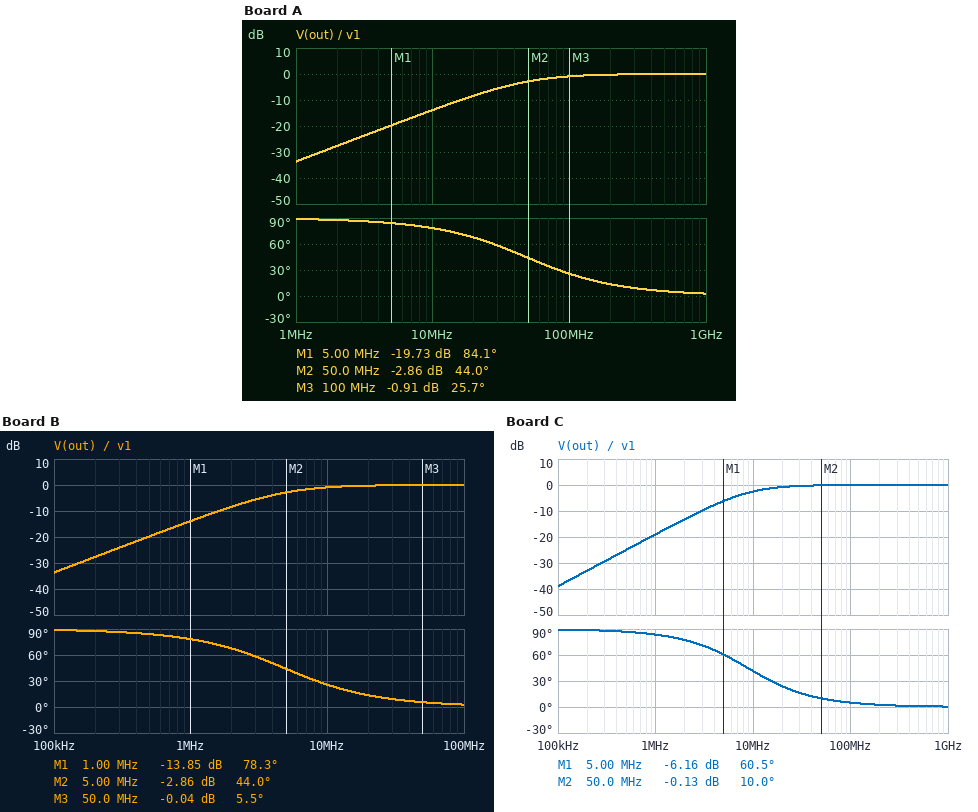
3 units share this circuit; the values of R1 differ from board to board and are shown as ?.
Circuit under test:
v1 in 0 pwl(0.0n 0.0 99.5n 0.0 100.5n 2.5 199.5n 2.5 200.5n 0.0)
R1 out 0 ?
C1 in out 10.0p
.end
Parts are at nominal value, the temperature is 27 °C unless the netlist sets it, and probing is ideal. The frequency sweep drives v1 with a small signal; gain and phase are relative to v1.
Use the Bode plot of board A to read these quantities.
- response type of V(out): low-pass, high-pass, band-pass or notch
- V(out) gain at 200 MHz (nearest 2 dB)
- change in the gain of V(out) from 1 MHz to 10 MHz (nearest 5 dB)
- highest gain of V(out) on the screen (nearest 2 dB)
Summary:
high-pass
0 dB
20 dB
0 dB
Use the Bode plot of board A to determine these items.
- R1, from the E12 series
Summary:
330 Ω
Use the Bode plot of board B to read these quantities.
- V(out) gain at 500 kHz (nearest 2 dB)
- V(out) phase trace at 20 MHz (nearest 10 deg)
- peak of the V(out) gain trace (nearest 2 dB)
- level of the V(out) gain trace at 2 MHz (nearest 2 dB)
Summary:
-20 dB
10 deg
0 dB
-8 dB
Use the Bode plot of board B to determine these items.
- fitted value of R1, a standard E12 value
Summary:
3.3 kΩ
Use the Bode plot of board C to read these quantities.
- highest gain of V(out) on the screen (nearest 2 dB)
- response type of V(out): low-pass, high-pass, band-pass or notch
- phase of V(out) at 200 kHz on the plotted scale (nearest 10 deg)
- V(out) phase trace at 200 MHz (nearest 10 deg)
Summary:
0 dB
high-pass
90 deg
0 deg
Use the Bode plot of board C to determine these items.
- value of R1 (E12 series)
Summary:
1.8 kΩ
